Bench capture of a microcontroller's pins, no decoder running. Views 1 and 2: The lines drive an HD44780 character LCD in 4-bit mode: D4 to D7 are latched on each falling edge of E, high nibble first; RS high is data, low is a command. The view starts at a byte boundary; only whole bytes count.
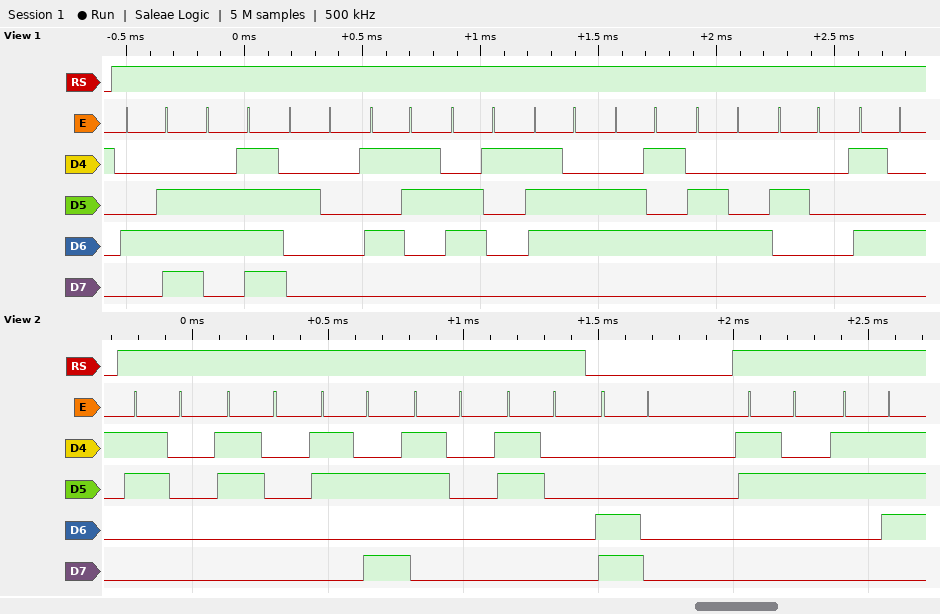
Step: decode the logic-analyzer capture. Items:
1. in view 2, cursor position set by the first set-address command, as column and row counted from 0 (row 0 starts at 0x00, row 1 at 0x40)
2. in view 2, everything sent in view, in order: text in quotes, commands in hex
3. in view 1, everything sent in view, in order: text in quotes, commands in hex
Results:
column 0, row 1
"00:00" 0xC0 "27"
"No Saved T"
